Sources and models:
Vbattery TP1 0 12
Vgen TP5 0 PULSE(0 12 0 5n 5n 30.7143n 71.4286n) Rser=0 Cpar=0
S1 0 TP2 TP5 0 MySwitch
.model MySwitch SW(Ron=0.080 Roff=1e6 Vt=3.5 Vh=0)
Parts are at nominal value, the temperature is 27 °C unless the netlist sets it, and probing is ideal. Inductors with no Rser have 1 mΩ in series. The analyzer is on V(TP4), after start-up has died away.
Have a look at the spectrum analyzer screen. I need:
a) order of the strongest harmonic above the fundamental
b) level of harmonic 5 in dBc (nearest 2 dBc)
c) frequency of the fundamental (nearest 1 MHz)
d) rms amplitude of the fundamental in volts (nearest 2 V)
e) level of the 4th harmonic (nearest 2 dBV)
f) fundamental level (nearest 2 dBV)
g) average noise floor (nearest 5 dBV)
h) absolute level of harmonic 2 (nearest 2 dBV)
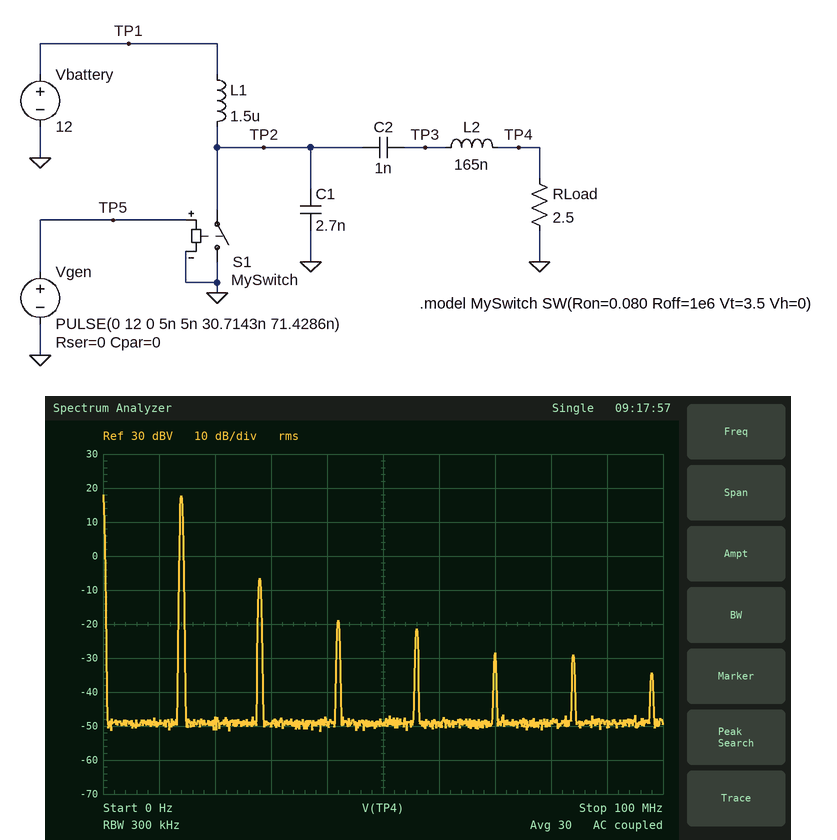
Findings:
2
-46 dBc
14 MHz
8 V
-22 dBV
18 dBV
-50 dBV
-6 dBV
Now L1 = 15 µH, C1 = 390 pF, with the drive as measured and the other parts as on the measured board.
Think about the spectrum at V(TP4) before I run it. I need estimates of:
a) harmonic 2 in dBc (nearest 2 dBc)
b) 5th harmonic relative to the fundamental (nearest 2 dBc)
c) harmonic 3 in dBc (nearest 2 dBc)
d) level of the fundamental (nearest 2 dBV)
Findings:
-16 dBc
-42 dBc
-26 dBc
20 dBV
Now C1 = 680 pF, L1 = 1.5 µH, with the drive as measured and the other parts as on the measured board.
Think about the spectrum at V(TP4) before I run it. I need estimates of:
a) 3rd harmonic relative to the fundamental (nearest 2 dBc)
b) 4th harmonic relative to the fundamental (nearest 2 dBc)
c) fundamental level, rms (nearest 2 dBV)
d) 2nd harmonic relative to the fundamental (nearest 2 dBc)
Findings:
-32 dBc
-46 dBc
20 dBV
-18 dBc
